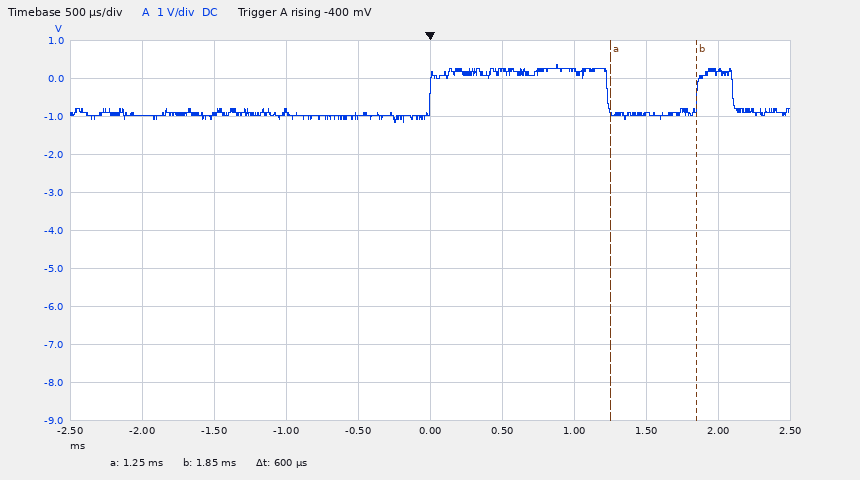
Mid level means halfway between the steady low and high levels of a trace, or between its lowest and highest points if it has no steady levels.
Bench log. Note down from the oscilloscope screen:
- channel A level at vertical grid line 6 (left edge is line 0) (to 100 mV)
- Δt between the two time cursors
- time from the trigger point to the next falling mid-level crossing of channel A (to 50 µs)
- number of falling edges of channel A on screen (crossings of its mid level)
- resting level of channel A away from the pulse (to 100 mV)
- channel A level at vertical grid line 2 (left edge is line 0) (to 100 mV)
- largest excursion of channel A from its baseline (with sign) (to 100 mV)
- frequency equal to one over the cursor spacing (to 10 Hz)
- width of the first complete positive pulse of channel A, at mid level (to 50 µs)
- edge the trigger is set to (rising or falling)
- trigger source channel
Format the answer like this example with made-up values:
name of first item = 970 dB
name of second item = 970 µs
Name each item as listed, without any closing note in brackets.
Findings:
channel A level at vertical grid line 6 (left edge is line 0) = 200 mV
Δt between the two time cursors = 600 µs
time from the trigger point to the next falling mid-level crossing of channel A = 1.25 ms
number of falling edges of channel A on screen = 2
resting level of channel A away from the pulse = -900 mV
channel A level at vertical grid line 2 (left edge is line 0) = -1.0 V
largest excursion of channel A from its baseline (with sign) = +1.3 V
frequency equal to one over the cursor spacing = 1.67 kHz
width of the first complete positive pulse of channel A, at mid level = 1.25 ms
edge the trigger is set to = rising
trigger source channel = channel A
